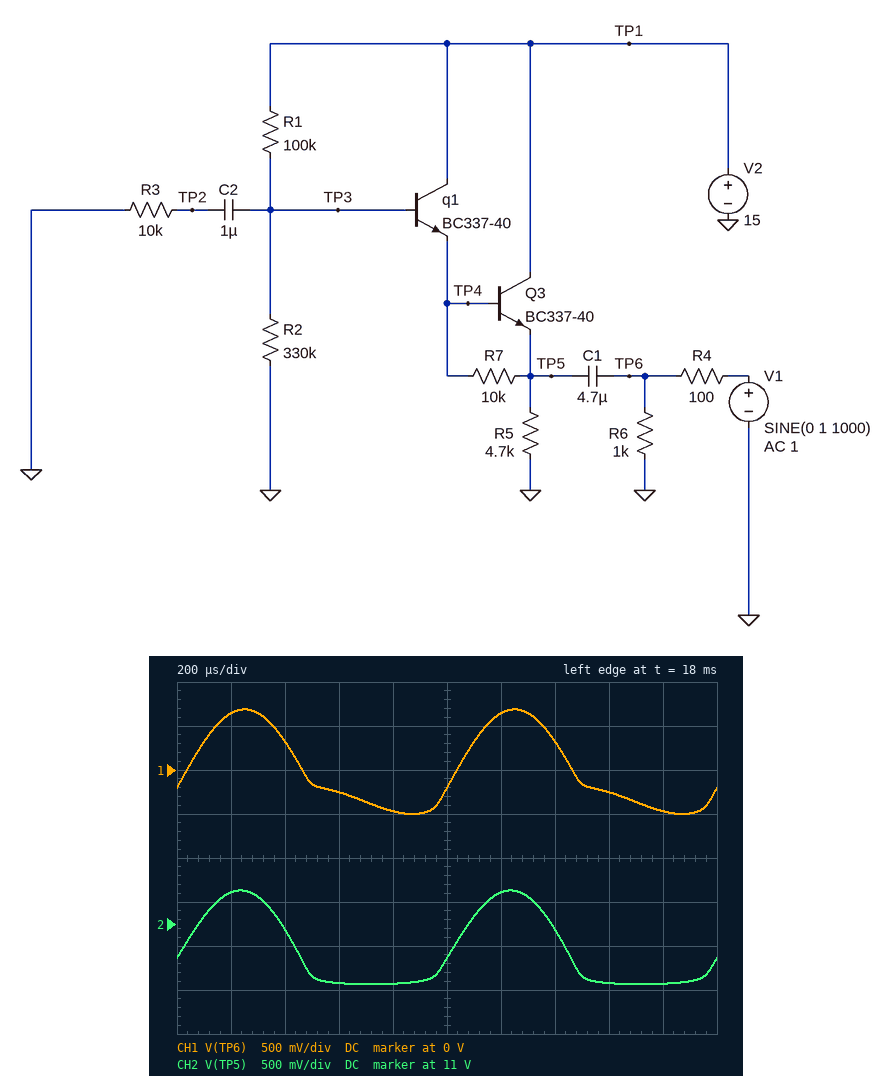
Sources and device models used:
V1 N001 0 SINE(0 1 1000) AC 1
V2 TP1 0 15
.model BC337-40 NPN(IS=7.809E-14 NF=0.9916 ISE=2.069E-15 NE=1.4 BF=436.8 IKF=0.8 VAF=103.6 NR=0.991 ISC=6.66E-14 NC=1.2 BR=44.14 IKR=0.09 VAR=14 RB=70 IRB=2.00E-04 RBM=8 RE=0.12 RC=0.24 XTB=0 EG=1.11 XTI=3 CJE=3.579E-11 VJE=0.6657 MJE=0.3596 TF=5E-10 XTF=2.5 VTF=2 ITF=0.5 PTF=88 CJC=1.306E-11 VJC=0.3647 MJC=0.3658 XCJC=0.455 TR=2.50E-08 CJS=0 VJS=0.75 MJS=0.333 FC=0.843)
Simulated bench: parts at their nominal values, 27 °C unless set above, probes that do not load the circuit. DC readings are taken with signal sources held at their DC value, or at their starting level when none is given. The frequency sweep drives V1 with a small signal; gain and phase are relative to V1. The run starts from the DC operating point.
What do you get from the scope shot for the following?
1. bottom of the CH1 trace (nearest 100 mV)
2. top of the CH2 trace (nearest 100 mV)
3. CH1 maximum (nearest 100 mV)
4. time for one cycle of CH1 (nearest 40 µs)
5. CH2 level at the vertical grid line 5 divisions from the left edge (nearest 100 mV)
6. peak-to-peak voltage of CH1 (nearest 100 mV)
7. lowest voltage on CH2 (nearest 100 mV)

-500 mV
11.4 V
700 mV
1.00 ms
10.6 V
1.2 V
10.3 V
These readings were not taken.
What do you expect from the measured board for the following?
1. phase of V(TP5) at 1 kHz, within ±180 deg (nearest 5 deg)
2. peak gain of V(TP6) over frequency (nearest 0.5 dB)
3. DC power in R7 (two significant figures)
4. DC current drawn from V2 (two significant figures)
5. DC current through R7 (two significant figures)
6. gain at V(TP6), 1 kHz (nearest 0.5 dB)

20 deg
-1.0 dB
38 µW
2.2 mA
62 µA
-10.5 dB
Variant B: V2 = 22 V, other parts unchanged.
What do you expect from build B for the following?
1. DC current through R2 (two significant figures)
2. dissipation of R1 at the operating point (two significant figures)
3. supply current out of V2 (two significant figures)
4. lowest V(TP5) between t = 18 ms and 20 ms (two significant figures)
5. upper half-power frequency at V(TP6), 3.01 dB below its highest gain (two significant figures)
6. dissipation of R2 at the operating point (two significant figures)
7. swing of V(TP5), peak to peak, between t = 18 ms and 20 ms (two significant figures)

51 µA
260 µW
3.4 mA
16 V
340 Hz
860 µW
850 mV
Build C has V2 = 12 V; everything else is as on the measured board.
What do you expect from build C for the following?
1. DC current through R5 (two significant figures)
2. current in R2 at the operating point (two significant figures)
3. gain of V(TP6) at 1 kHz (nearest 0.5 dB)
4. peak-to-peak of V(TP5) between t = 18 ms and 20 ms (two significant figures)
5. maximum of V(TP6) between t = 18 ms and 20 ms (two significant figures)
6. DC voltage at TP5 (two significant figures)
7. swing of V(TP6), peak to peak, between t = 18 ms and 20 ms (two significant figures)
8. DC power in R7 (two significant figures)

1.7 mA
28 µA
-10.5 dB
1.2 V
730 mV
8.1 V
1.3 V
37 µW
